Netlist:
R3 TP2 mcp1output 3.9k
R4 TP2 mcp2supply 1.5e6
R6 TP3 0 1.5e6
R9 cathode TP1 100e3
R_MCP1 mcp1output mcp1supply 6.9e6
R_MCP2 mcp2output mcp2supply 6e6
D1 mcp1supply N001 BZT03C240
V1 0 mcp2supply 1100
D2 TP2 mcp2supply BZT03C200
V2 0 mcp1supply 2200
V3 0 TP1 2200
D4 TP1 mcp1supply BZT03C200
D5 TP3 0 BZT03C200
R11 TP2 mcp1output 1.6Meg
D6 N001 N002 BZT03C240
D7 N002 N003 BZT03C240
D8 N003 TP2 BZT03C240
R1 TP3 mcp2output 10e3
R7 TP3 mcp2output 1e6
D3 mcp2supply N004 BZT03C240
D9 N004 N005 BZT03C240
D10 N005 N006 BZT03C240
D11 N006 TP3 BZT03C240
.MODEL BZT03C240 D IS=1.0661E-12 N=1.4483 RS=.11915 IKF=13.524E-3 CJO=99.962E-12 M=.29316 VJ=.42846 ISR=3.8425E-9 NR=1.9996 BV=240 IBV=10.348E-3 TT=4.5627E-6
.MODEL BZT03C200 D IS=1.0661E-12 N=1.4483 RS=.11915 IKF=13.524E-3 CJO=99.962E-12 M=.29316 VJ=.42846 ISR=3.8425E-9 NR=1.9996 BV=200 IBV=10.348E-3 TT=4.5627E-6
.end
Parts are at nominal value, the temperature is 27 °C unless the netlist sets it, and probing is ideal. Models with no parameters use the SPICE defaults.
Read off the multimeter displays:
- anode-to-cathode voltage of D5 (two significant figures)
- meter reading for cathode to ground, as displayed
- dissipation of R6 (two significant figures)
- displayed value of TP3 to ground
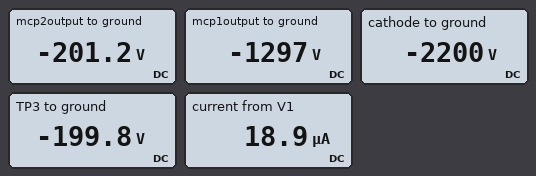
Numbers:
-200 V
-2200 V
27 mW
-199.8 V
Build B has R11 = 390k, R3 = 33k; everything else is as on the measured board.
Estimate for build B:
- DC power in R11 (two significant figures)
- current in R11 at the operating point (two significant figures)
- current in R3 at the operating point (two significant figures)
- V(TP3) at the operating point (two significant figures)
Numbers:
40 µW
10 µA
120 µA
-200 V
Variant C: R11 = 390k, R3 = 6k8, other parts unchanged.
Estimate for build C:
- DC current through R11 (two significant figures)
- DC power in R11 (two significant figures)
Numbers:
2.2 µA
2.0 µW
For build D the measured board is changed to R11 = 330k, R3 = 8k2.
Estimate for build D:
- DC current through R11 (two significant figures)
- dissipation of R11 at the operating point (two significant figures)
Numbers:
3.2 µA
3.3 µW
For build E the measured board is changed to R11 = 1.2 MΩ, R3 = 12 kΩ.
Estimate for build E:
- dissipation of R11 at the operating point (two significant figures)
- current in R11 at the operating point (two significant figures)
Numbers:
2.0 µW
1.3 µA
